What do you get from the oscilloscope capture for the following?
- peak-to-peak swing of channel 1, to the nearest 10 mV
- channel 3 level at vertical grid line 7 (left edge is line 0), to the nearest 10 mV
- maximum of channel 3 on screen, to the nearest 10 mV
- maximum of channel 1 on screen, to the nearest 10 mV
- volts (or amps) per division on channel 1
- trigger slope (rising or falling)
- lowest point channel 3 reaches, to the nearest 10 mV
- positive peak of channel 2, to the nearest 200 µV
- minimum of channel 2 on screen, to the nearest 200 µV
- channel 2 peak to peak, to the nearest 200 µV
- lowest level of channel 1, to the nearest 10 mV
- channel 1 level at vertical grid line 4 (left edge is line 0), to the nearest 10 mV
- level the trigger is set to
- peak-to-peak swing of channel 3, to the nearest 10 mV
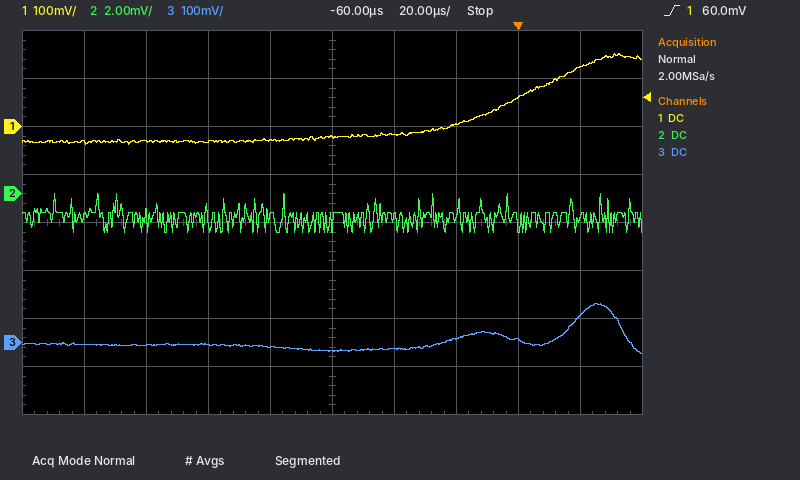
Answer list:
190 mV
10 mV
80 mV
150 mV
100 mV
rising
-20 mV
0.0 mV
-1.6 mV
1.6 mV
-40 mV
-30 mV
60.0 mV
100 mV
